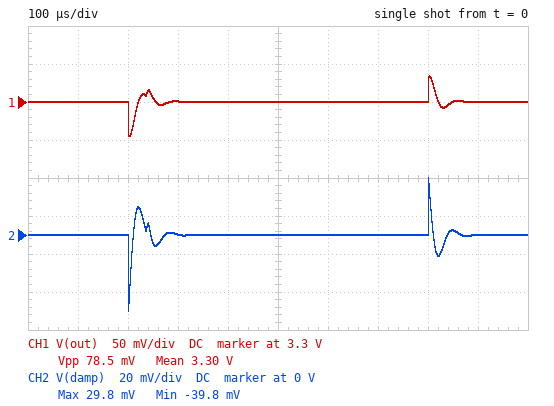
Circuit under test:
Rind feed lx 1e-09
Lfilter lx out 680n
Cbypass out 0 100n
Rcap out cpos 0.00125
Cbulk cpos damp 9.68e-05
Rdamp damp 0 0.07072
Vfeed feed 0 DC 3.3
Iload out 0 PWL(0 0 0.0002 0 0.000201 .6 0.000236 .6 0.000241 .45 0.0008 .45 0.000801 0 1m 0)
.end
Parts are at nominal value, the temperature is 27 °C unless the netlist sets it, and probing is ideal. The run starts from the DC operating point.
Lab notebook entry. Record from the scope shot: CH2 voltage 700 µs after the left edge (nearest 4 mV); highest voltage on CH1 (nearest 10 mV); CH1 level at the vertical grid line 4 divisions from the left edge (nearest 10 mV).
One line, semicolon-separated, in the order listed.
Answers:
0 V; 3.33 V; 3.30 V
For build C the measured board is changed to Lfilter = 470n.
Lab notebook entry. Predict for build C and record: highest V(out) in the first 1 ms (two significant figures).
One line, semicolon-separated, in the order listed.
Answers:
3.3 V
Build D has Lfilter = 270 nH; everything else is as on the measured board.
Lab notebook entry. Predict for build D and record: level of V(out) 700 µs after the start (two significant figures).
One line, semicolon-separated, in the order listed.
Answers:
3.3 V
